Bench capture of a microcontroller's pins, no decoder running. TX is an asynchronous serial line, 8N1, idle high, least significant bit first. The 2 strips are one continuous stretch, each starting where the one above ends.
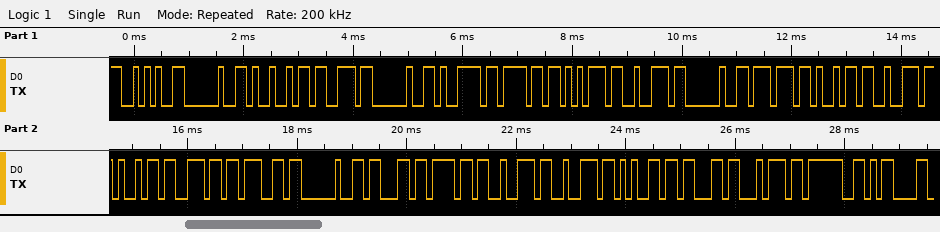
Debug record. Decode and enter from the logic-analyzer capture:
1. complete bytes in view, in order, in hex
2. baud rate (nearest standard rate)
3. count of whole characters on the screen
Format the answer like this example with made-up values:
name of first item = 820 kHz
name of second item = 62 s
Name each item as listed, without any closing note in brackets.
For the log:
complete bytes in view, in order, in hex = 2A 20 49 73 20 79 6F 75 72 20 77 69 72 69 6E 67 20 63 6F 72 72 65 63 74 3F 0D
baud rate = 9600 baud
count of whole characters on the screen = 26
